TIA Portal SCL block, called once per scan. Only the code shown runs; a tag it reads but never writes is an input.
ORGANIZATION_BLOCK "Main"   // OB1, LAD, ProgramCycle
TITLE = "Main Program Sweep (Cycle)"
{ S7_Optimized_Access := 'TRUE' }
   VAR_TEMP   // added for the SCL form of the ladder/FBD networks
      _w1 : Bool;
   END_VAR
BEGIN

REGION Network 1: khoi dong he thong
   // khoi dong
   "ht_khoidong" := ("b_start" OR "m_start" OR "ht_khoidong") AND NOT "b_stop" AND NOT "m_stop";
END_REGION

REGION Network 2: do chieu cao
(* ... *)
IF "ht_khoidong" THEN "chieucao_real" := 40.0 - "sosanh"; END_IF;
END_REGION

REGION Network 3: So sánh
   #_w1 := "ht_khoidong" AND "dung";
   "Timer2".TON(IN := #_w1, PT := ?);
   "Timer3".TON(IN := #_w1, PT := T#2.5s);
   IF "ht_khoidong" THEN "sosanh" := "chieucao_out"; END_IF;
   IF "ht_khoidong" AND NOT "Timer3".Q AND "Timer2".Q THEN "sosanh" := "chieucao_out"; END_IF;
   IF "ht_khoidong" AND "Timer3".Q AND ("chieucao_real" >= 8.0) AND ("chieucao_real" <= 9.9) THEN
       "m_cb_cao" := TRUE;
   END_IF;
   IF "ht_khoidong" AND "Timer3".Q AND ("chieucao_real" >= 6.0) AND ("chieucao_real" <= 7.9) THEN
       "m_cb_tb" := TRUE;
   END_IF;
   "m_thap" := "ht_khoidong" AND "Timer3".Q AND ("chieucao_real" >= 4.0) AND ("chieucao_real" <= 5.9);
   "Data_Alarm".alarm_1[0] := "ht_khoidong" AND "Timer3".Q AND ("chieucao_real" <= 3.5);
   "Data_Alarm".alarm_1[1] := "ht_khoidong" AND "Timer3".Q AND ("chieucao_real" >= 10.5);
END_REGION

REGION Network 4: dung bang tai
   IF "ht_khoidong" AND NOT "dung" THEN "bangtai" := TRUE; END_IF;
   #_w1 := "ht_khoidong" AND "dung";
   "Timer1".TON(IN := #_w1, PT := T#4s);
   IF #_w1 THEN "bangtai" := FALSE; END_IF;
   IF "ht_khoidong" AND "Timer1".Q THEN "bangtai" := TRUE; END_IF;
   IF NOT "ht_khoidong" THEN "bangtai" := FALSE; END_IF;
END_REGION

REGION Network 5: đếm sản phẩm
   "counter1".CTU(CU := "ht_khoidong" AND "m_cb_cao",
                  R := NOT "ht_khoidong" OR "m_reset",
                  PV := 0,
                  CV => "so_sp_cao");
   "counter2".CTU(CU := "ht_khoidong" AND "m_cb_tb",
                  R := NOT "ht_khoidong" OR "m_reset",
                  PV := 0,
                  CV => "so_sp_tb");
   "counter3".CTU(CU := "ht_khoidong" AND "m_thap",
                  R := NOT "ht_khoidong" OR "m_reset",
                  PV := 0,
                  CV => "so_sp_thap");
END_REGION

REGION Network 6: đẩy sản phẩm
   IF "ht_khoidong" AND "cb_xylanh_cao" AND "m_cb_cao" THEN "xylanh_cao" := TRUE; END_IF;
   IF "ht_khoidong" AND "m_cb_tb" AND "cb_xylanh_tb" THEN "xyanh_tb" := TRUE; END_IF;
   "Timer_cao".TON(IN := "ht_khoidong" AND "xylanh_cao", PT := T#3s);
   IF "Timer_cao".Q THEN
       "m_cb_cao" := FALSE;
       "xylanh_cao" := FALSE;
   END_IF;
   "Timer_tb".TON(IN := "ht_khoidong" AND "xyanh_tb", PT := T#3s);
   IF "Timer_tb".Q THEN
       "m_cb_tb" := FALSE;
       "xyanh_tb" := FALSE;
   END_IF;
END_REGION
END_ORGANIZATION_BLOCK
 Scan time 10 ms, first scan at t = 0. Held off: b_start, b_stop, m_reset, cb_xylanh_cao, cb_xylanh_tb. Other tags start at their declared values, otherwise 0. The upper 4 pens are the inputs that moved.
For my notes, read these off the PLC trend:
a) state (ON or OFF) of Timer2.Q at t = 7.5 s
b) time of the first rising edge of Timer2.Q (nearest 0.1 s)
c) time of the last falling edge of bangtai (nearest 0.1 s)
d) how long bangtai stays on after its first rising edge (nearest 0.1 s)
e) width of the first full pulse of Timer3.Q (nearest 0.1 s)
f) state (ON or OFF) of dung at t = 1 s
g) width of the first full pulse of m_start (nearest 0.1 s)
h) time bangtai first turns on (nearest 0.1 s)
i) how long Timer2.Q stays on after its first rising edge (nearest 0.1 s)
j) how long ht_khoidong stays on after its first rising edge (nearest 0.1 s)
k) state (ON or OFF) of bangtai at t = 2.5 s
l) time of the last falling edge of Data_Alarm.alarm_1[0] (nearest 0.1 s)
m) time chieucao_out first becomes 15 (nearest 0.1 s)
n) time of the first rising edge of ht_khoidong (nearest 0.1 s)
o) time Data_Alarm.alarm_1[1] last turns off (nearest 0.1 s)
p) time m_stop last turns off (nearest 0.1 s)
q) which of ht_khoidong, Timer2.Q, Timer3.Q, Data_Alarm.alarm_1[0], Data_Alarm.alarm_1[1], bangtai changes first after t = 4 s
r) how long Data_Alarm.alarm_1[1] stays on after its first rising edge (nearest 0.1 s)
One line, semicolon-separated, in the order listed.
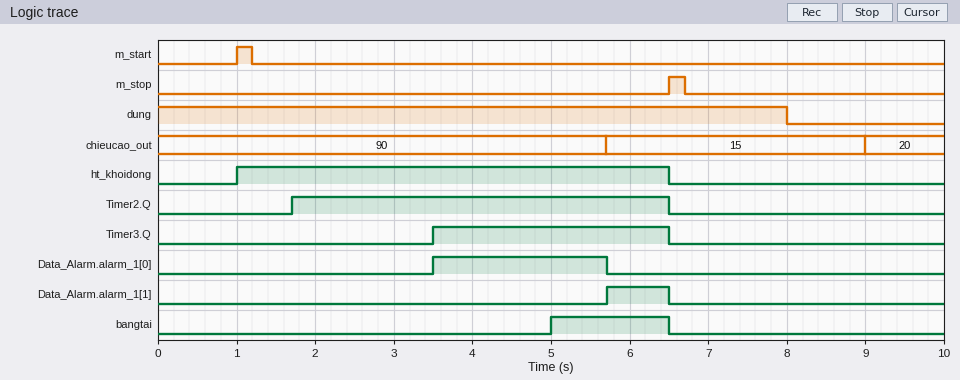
OFF; 1.7 s; 6.5 s; 1.5 s; 3.0 s; ON; 0.2 s; 5.0 s; 4.8 s; 5.5 s; OFF; 5.7 s; 5.7 s; 1.0 s; 6.5 s; 6.7 s; bangtai; 0.8 s
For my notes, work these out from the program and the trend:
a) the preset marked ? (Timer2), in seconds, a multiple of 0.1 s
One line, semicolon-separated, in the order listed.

0.7 s
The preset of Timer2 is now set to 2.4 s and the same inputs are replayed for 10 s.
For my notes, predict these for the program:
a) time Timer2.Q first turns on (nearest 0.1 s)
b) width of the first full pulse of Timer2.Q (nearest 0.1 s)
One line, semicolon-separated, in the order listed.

3.4 s; 3.1 s
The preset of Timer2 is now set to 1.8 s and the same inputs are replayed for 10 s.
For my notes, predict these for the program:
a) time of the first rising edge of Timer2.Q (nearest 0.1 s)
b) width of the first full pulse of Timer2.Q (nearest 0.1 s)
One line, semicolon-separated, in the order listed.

2.8 s; 3.7 s
